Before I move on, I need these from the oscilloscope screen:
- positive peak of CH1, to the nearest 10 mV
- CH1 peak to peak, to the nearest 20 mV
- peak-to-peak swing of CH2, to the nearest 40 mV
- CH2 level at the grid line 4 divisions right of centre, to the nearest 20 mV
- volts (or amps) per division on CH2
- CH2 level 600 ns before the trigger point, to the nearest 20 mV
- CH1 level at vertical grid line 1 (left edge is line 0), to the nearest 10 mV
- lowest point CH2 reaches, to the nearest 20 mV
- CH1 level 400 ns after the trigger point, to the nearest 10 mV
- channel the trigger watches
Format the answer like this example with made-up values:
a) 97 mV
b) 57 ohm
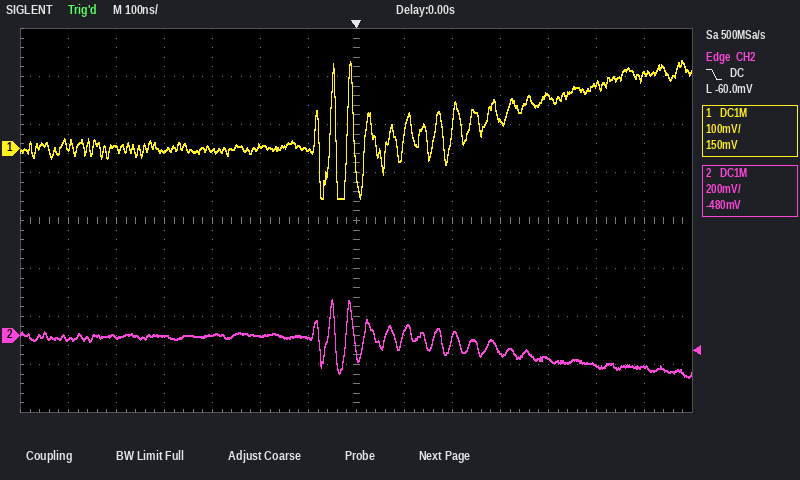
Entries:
a) 180 mV
b) 280 mV
c) 320 mV
d) -100 mV
e) 200 mV
f) -20 mV
g) 0 mV
h) -180 mV
i) 110 mV
j) CH2
